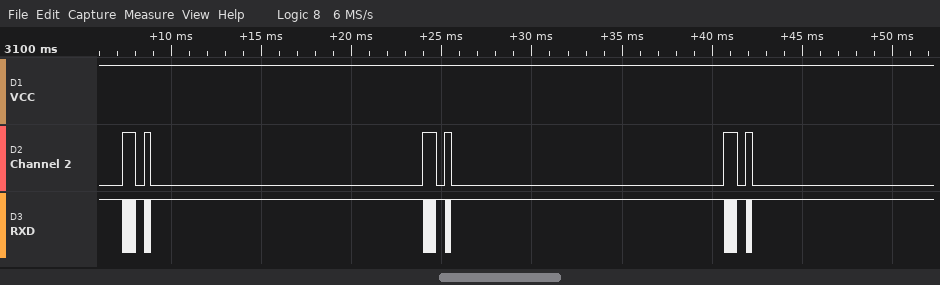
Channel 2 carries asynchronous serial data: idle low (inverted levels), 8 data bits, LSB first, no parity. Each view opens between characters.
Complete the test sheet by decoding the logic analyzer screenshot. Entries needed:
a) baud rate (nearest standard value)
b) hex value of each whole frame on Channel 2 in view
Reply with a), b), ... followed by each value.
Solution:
a) 2400 baud
b) FA, FA, FA
